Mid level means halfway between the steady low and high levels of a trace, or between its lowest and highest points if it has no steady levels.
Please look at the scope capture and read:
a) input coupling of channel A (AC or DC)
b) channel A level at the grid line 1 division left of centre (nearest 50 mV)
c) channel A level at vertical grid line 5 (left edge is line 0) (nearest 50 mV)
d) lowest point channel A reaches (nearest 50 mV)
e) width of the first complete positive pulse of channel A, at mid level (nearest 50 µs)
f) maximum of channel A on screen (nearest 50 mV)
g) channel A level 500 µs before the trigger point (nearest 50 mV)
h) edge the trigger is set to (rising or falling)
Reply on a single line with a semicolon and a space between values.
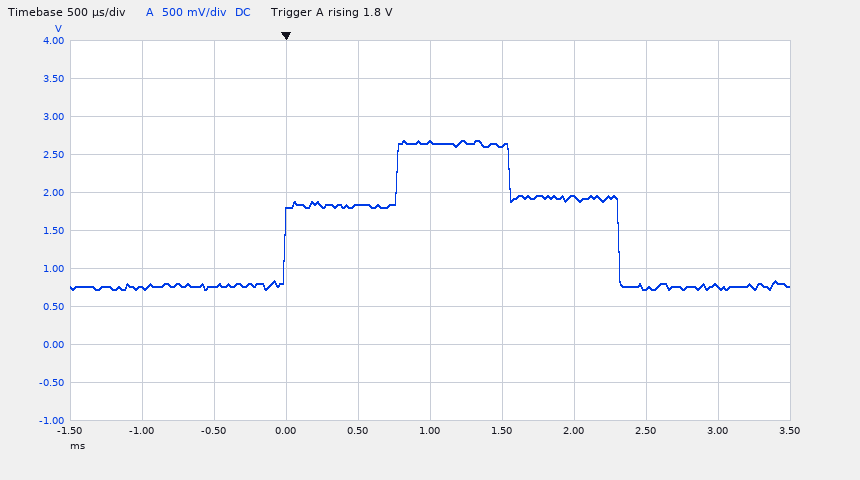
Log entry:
DC; 1.85 V; 2.65 V; 700 mV; 2.30 ms; 2.70 V; 750 mV; rising
